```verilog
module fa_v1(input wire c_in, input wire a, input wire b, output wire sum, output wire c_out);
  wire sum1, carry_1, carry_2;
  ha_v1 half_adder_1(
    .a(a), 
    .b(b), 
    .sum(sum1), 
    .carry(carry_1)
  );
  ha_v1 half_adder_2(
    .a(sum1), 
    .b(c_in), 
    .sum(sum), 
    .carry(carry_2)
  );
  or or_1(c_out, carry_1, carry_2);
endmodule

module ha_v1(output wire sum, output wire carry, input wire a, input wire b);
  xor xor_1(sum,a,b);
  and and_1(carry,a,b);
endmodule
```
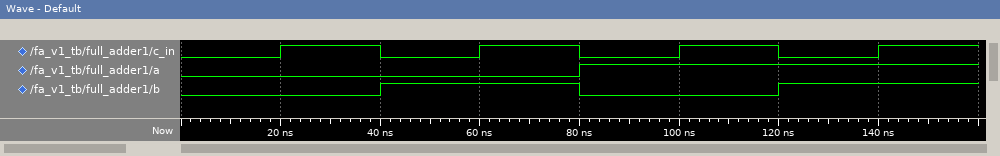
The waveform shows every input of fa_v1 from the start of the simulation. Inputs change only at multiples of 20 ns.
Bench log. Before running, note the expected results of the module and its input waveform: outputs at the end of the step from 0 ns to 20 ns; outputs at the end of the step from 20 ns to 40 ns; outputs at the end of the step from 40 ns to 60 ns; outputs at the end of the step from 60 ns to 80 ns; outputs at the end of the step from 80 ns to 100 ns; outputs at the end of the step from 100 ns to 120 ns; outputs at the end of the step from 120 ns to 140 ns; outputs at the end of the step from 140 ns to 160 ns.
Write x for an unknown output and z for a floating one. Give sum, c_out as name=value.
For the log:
sum=0, c_out=0
sum=1, c_out=0
sum=1, c_out=0
sum=0, c_out=1
sum=1, c_out=0
sum=0, c_out=1
sum=0, c_out=1
sum=1, c_out=1
